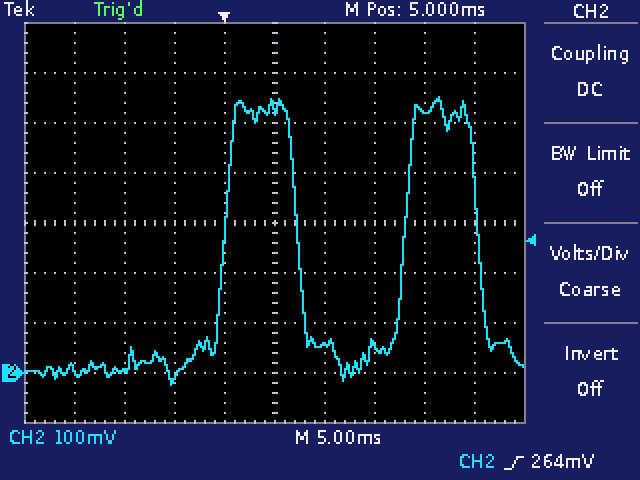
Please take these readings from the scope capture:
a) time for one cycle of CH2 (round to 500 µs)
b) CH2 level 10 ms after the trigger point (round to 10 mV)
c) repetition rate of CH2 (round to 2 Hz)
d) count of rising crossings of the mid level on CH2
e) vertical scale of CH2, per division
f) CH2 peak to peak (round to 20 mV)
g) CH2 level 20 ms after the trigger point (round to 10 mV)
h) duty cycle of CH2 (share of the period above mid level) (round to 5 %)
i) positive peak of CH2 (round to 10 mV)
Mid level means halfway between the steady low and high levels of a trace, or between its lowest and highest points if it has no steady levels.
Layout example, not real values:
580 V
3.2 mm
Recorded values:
18.0 ms
60 mV
56 Hz
2
100 mV
580 mV
520 mV
40 %
550 mV
